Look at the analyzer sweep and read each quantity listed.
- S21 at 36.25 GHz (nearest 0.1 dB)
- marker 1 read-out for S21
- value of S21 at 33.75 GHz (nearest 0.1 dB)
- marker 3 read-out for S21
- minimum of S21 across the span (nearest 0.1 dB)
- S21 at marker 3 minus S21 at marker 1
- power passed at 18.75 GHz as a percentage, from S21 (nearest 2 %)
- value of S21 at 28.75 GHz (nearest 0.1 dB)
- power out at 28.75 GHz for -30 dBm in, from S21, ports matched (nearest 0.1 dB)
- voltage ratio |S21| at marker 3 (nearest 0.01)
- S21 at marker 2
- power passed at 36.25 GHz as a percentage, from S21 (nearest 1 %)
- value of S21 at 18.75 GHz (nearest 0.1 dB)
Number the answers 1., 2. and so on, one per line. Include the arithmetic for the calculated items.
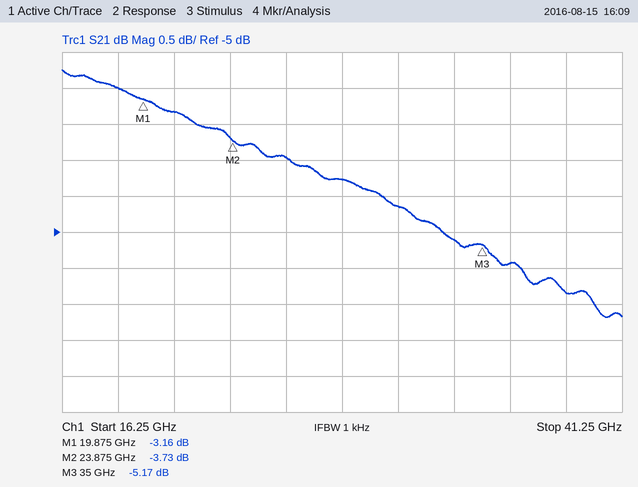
1. -5.4 dB
2. -3.16 dB
3. -5.1 dB
4. -5.17 dB
5. -6.2 dB
6. -5.17 − (-3.16) = -2.01 dB
7. 10^(-3/10) ≈ 50 %
8. -4.3 dB
9. -30 dBm + (-4.3 dB) = -34.3 dBm
10. 10^(-5.17/20) ≈ 0.55
11. -3.73 dB
12. 10^(-5.4/10) ≈ 29 %
13. -3.0 dB
